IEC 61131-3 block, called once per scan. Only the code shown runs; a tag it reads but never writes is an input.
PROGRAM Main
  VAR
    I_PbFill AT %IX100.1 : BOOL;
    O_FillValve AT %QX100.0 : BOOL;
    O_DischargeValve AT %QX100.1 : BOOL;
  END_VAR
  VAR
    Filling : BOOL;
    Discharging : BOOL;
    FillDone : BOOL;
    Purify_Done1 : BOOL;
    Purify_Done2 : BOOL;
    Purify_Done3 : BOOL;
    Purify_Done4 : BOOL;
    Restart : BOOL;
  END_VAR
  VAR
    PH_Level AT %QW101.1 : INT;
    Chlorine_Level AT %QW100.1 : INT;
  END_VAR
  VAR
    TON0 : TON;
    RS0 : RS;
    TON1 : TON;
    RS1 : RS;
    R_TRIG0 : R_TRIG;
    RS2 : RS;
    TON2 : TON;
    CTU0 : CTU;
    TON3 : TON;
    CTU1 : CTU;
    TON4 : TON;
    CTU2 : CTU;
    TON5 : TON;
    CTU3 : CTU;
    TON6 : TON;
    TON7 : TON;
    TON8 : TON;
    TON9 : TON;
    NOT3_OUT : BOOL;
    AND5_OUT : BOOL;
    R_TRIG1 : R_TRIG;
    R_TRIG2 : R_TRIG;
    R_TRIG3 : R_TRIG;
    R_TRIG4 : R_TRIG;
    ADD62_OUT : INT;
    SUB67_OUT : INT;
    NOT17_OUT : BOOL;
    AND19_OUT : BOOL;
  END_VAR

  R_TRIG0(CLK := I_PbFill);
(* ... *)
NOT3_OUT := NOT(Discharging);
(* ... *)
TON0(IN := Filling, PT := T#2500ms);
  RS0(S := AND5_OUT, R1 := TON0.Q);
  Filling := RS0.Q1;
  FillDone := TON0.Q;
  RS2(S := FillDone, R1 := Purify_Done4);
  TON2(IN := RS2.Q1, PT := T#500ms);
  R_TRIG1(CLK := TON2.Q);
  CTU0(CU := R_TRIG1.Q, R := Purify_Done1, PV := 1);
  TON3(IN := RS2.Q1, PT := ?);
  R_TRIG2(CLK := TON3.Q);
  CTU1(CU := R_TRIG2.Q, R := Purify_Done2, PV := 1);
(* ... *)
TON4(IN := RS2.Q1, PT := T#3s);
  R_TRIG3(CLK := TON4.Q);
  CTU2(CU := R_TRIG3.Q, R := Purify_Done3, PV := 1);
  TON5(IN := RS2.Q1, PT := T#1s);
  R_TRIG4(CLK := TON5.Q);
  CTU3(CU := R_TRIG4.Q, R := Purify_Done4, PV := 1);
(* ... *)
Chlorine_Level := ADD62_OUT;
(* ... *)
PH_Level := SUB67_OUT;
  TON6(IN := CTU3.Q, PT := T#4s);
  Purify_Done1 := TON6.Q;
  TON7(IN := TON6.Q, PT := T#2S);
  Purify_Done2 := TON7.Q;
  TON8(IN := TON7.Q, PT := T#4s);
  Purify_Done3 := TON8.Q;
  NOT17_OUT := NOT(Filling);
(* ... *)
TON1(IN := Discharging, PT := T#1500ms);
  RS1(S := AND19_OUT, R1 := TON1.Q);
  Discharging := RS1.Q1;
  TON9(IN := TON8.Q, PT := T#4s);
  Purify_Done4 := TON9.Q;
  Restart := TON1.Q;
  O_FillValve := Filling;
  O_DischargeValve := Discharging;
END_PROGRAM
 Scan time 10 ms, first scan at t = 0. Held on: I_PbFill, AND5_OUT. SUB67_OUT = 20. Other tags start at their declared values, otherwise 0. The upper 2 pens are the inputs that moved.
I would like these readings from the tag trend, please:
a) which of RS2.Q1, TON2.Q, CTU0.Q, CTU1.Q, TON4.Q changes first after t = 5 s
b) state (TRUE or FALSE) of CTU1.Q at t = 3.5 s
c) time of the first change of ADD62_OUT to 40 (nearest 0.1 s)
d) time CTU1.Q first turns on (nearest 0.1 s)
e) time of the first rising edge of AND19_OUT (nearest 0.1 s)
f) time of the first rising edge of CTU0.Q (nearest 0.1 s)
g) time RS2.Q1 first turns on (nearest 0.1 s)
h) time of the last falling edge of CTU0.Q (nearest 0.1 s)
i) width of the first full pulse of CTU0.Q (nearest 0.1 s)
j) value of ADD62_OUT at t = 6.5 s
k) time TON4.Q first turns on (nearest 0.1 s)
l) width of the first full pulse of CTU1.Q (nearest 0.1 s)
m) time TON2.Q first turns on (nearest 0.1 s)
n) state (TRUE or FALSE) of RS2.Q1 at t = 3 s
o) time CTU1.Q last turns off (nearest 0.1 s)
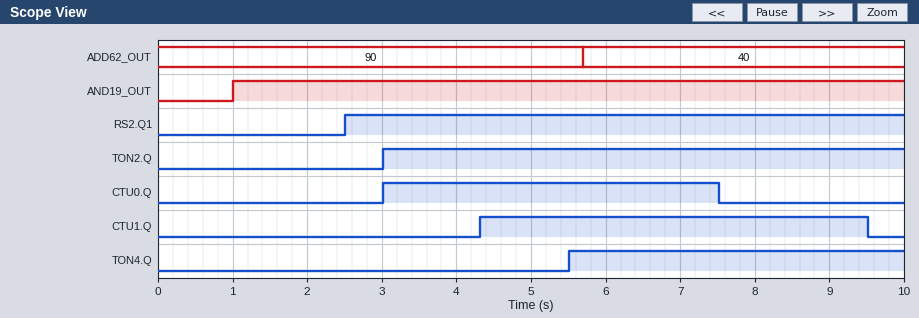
TON4.Q
FALSE
5.7 s
4.3 s
1.0 s
3.0 s
2.5 s
7.5 s
4.5 s
40
5.5 s
5.2 s
3.0 s
TRUE
9.5 s
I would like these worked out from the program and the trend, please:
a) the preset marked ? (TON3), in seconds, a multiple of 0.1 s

1.8 s
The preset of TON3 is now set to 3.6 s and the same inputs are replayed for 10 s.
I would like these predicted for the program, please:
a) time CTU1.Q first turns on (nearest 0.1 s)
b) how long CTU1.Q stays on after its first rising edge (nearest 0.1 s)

6.1 s
3.4 s
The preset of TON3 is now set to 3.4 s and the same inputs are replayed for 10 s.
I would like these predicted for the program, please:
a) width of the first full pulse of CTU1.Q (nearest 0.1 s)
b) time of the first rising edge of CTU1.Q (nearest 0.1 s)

3.6 s
5.9 s
